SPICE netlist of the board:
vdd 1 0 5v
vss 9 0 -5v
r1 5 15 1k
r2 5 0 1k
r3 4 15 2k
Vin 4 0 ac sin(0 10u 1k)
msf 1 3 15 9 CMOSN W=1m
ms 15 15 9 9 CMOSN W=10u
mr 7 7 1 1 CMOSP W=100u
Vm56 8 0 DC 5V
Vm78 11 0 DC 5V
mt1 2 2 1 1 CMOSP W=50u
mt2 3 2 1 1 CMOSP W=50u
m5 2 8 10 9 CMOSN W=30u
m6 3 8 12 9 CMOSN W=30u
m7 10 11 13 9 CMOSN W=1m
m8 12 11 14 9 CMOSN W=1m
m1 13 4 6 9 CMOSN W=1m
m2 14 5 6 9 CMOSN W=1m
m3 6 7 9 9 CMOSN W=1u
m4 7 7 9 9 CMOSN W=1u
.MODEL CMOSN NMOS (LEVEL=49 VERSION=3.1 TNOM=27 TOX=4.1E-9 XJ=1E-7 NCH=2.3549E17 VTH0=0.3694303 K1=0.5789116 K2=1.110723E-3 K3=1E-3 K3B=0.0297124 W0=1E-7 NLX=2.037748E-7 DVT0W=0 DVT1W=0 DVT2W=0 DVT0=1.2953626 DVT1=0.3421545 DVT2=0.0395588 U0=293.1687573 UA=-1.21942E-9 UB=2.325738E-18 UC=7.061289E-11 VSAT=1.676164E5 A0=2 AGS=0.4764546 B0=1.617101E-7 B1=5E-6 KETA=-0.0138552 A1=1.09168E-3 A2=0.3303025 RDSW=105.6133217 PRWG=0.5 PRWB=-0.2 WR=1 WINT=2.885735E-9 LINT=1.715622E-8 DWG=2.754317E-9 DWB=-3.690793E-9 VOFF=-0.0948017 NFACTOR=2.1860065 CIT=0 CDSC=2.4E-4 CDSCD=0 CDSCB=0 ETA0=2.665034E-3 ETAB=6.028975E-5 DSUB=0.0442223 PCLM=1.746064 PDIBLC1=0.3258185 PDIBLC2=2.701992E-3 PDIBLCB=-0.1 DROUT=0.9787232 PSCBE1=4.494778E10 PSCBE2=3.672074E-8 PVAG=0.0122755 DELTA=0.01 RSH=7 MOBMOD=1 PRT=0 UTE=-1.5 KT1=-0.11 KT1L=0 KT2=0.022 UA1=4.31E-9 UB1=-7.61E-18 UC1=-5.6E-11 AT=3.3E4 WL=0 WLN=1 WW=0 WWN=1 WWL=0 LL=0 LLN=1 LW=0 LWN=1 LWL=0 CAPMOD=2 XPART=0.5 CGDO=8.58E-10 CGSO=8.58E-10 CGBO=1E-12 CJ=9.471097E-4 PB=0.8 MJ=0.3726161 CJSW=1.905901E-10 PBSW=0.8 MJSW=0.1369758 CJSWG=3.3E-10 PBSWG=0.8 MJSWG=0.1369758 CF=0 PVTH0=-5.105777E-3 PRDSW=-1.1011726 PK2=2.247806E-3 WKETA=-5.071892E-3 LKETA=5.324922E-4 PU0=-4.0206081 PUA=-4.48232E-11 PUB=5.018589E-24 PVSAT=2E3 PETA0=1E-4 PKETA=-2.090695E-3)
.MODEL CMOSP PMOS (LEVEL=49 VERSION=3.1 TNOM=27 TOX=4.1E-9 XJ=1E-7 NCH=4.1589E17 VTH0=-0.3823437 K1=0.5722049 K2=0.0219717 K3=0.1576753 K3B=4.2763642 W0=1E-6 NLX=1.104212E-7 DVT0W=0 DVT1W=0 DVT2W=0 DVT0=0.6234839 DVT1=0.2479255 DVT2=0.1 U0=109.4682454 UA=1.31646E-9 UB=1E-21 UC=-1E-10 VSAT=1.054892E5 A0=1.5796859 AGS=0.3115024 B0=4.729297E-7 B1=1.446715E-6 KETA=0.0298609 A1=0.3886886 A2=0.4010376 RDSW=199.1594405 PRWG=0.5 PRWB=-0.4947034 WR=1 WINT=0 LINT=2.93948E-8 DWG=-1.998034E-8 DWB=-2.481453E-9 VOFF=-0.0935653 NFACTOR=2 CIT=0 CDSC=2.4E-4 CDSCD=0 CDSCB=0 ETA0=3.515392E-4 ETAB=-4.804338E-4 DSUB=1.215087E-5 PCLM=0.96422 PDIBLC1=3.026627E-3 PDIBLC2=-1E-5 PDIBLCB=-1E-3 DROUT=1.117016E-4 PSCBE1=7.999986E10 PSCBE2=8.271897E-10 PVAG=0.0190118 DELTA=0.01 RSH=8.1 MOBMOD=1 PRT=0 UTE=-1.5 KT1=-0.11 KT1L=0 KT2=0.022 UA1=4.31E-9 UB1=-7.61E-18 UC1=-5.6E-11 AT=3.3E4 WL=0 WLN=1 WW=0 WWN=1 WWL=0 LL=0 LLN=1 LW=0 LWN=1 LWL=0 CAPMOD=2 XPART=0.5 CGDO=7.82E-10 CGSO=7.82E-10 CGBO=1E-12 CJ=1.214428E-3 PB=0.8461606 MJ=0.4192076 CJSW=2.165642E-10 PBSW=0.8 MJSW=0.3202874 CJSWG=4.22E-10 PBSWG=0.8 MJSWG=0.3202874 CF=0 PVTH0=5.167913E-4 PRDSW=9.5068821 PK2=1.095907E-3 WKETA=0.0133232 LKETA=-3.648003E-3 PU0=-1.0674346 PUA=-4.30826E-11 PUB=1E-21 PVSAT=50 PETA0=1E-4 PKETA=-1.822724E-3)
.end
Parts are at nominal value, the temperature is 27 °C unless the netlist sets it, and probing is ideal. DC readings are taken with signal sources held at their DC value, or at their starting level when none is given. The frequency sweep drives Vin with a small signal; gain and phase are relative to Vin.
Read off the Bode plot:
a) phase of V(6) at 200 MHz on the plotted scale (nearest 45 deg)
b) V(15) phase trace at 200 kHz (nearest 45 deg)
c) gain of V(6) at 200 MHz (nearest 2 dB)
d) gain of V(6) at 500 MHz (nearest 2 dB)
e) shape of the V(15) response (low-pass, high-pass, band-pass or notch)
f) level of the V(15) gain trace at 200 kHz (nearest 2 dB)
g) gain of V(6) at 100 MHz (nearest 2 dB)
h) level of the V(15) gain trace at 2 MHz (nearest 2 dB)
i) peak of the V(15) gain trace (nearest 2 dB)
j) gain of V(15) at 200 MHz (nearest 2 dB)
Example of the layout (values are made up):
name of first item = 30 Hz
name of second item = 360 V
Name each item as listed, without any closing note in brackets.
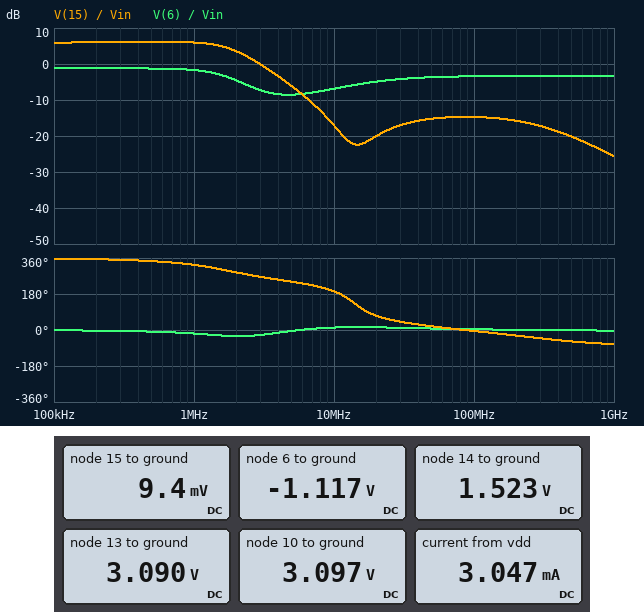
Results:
phase of V(6) at 200 MHz on the plotted scale = 0 deg
V(15) phase trace at 200 kHz = 360 deg
gain of V(6) at 200 MHz = -4 dB
gain of V(6) at 500 MHz = -4 dB
shape of the V(15) response = low-pass
level of the V(15) gain trace at 200 kHz = 6 dB
gain of V(6) at 100 MHz = -4 dB
level of the V(15) gain trace at 2 MHz = 4 dB
peak of the V(15) gain trace = 6 dB
gain of V(15) at 200 MHz = -16 dB
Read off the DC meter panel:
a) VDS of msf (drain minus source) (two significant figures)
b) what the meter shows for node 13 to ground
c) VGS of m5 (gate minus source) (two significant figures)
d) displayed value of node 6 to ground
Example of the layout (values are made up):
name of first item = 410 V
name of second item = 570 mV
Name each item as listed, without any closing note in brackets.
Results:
VDS of msf (drain minus source) = 5.0 V
what the meter shows for node 13 to ground = 3.090 V
VGS of m5 (gate minus source) = 1.9 V
displayed value of node 6 to ground = -1.117 V
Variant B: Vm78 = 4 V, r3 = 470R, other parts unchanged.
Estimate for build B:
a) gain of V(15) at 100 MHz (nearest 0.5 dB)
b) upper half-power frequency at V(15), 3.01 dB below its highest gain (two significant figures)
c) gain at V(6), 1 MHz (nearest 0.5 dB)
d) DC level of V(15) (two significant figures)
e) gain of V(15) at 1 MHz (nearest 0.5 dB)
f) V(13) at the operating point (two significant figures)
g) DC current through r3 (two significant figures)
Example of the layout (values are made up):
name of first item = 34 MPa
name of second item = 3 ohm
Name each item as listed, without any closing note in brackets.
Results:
gain of V(15) at 100 MHz = -9.5 dB
upper half-power frequency at V(15), 3.01 dB below its highest gain = 2.0 MHz
gain at V(6), 1 MHz = -2.0 dB
DC level of V(15) = 7.1 mV
gain of V(15) at 1 MHz = 5.0 dB
V(13) at the operating point = 2.5 V
DC current through r3 = 15 µA
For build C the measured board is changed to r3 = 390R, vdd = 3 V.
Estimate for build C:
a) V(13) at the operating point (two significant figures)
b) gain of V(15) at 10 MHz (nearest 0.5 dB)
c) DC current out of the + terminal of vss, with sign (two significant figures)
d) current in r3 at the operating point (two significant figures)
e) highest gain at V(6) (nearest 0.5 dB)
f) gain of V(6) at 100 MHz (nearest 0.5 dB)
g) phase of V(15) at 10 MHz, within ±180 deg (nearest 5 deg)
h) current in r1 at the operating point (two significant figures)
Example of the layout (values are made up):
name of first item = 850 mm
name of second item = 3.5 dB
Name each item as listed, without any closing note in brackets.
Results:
V(13) at the operating point = 1.9 V
gain of V(15) at 10 MHz = -23.0 dB
DC current out of the + terminal of vss, with sign = -3.1 mA
current in r3 at the operating point = 5.6 µA
highest gain at V(6) = -1.0 dB
gain of V(6) at 100 MHz = -3.0 dB
phase of V(15) at 10 MHz, within ±180 deg = 5 deg
current in r1 at the operating point = 1.1 µA
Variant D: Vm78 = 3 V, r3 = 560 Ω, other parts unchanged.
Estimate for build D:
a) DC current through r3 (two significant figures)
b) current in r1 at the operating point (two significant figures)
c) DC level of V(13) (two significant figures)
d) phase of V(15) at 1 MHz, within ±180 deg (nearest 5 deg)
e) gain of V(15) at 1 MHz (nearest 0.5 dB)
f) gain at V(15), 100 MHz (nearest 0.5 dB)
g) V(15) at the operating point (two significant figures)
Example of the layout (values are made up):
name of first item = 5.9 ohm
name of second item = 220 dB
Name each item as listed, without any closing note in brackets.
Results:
DC current through r3 = 6.8 µA
current in r1 at the operating point = 1.9 µA
DC level of V(13) = 1.6 V
phase of V(15) at 1 MHz, within ±180 deg = -25 deg
gain of V(15) at 1 MHz = 5.5 dB
gain at V(15), 100 MHz = -10.0 dB
V(15) at the operating point = 3.8 mV
